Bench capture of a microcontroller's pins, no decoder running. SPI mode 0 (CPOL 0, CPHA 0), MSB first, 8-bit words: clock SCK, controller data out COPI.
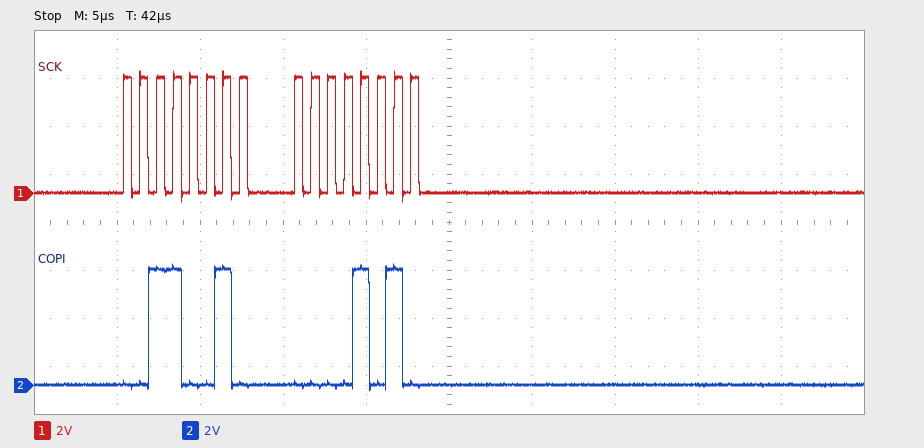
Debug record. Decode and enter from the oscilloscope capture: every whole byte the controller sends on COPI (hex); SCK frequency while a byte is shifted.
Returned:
32 0A
1 MHz
